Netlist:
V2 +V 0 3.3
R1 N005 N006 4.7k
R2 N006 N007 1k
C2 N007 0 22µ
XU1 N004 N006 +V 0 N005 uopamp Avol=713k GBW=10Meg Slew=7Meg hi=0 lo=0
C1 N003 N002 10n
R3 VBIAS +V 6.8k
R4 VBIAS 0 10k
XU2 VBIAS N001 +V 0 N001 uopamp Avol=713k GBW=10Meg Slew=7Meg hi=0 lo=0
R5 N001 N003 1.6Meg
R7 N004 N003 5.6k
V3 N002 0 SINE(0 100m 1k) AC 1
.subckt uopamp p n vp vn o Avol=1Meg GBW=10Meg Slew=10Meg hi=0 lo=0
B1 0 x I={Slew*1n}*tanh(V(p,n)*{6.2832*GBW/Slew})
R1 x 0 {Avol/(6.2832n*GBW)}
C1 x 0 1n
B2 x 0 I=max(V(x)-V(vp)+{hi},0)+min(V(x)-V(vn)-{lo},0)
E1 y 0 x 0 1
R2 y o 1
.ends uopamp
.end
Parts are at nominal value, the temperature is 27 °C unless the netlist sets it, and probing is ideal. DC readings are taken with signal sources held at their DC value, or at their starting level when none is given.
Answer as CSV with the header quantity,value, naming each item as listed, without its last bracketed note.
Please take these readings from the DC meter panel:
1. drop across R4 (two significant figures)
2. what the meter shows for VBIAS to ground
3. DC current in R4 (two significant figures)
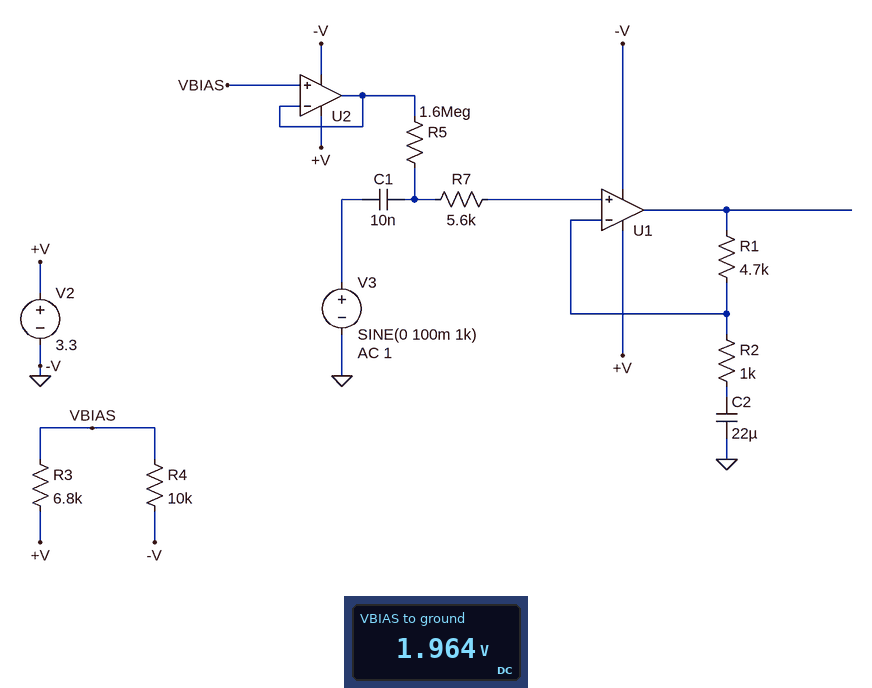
quantity,value
drop across R4,2.0 V
what the meter shows for VBIAS to ground,1.964 V
DC current in R4,200 µA
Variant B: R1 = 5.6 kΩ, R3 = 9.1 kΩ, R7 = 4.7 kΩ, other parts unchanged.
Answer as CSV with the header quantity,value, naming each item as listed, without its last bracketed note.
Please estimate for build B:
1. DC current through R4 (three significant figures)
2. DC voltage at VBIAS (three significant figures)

quantity,value
DC current through R4,173 µA
DC voltage at VBIAS,1.73 V
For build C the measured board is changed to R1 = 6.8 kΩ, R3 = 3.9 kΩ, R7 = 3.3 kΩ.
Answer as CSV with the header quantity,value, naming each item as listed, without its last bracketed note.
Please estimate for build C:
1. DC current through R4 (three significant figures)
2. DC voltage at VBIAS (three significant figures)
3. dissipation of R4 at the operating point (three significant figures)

quantity,value
DC current through R4,237 µA
DC voltage at VBIAS,2.37 V
dissipation of R4 at the operating point,564 µW
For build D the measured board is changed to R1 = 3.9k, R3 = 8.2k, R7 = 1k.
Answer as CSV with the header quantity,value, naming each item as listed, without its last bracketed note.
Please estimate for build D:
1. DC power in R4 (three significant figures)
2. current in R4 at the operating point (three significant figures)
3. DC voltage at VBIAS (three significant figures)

quantity,value
DC power in R4,329 µW
current in R4 at the operating point,181 µA
DC voltage at VBIAS,1.81 V
